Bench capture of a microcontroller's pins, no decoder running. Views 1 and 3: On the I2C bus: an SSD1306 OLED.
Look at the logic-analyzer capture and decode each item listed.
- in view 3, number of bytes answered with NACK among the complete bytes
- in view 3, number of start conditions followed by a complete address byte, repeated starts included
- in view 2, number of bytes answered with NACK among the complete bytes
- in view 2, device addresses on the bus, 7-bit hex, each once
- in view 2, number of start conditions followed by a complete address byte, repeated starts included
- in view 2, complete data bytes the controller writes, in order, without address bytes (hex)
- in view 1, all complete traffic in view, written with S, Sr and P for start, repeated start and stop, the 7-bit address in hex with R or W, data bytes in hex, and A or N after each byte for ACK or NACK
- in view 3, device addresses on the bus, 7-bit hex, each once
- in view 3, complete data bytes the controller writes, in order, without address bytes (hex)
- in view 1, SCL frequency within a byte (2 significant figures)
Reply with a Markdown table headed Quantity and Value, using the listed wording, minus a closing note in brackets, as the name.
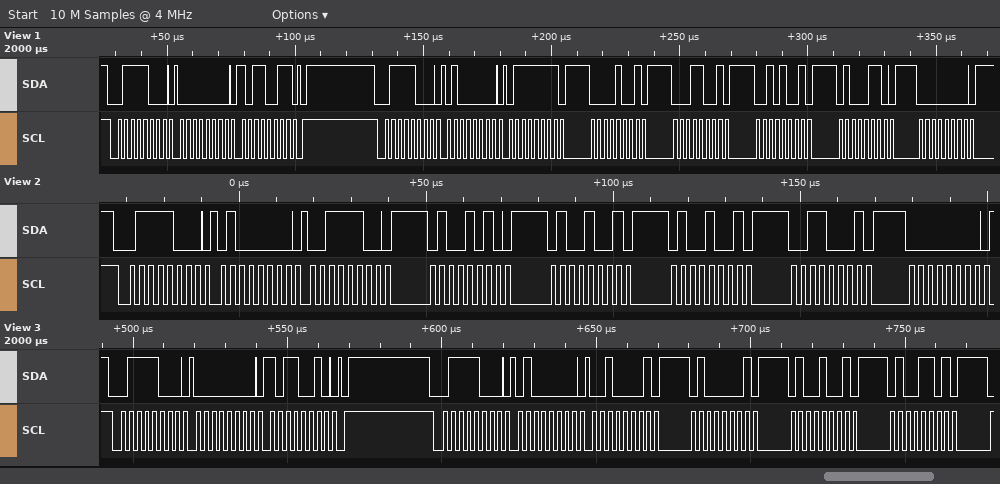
| Quantity | Value |
|---|---|
| in view 3, number of bytes answered with NACK among the complete bytes | 0 |
| in view 3, number of start conditions followed by a complete address byte, repeated starts included | 2 |
| in view 2, number of bytes answered with NACK among the complete bytes | 0 |
| in view 2, device addresses on the bus, 7-bit hex, each once | 0x3C |
| in view 2, number of start conditions followed by a complete address byte, repeated starts included | 1 |
| in view 2, complete data bytes the controller writes, in order, without address bytes | 40 3C 4A 49 49 31 00 |
| in view 1, all complete traffic in view, written with S, Sr and P for start, repeated start and stop, the 7-bit address in hex with R or W, data bytes in hex, and A or N after each byte for ACK or NACK | S 3CW A 00 A B3 A P S 3CW A 40 A 7F A 09 A 19 A 29 A 46 A 00 A |
| in view 3, device addresses on the bus, 7-bit hex, each once | 0x3C |
| in view 3, complete data bytes the controller writes, in order, without address bytes | 00 B2 40 21 41 49 4D |
| in view 1, SCL frequency within a byte | 400 kHz |
